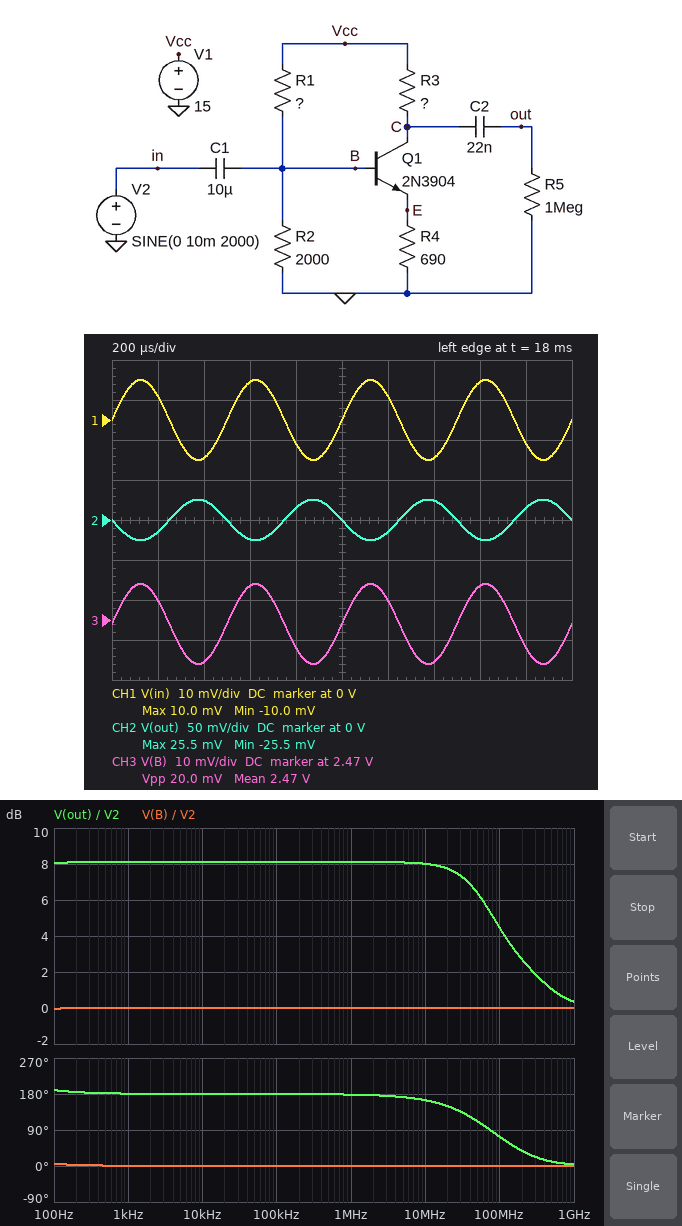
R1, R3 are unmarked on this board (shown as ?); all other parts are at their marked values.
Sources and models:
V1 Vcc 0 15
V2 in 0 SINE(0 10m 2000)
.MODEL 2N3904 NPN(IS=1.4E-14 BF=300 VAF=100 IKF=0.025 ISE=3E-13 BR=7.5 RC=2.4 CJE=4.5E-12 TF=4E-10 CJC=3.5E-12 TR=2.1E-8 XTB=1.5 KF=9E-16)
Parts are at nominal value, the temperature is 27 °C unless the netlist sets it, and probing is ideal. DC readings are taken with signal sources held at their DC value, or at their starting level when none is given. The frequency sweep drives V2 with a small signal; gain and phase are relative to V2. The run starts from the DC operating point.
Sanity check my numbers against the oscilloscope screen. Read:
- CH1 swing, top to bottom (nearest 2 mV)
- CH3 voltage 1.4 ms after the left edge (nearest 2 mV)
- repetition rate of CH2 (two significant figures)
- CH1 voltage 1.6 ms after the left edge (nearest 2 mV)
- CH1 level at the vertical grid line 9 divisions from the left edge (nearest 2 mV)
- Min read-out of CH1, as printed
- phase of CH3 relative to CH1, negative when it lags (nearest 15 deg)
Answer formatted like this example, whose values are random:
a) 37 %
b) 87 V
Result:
a) 20 mV
b) 2.460 V
c) 2.0 kHz
d) 10 mV
e) -6 mV
f) -10.0 mV
g) 0 deg
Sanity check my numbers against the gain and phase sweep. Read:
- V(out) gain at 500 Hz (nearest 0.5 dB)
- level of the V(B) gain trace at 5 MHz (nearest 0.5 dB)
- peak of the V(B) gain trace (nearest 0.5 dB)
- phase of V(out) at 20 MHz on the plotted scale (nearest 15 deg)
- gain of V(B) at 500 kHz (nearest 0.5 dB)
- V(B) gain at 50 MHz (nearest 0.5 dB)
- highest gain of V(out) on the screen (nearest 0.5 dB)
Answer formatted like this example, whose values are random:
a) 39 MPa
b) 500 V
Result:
a) 8.0 dB
b) 0 dB
c) 0 dB
d) 150 deg
e) 0 dB
f) 0 dB
g) 8.0 dB
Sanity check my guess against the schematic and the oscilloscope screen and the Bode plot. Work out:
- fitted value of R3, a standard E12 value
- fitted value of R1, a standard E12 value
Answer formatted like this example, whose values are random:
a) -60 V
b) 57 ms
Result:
a) 1.8 kΩ
b) 10 kΩ
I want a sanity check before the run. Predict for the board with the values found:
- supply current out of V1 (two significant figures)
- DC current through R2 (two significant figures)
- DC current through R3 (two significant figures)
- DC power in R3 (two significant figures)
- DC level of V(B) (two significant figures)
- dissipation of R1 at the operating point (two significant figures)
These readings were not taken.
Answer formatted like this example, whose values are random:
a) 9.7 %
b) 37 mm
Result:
a) 3.8 mA
b) 1.2 mA
c) 2.6 mA
d) 12 mW
e) 2.5 V
f) 16 mW
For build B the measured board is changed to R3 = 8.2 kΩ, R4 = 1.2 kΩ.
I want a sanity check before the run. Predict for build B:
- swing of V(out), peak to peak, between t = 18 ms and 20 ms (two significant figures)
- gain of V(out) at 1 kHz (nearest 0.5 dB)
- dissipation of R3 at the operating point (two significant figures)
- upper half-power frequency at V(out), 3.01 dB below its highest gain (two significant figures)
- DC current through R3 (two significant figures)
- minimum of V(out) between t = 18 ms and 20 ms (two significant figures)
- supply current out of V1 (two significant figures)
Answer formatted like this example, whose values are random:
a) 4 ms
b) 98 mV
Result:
a) 130 mV
b) 16.5 dB
c) 19 mW
d) 6.2 MHz
e) 1.5 mA
f) -66 mV
g) 2.8 mA
